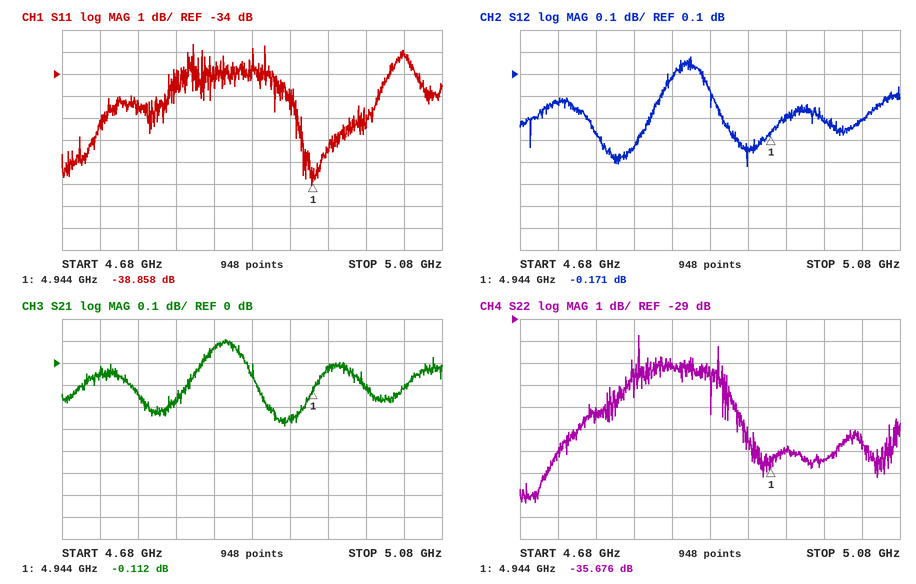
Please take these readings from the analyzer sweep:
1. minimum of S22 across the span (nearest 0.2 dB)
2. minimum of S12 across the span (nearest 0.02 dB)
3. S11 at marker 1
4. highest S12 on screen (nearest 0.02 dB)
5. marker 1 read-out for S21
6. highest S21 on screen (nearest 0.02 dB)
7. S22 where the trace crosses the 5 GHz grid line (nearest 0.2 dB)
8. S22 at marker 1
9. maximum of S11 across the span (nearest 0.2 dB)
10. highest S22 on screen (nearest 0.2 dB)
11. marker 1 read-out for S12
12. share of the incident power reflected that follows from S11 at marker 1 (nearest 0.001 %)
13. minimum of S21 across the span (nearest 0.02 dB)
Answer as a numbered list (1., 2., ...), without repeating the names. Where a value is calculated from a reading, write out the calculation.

1. -37.4 dB
2. -0.32 dB
3. -38.858 dB
4. 0.18 dB
5. -0.112 dB
6. 0.10 dB
7. -35.4 dB
8. -35.676 dB
9. -32.6 dB
10. -29.8 dB
11. -0.171 dB
12. 10^(-38.858/10) ≈ 0.013 %
13. -0.28 dB
